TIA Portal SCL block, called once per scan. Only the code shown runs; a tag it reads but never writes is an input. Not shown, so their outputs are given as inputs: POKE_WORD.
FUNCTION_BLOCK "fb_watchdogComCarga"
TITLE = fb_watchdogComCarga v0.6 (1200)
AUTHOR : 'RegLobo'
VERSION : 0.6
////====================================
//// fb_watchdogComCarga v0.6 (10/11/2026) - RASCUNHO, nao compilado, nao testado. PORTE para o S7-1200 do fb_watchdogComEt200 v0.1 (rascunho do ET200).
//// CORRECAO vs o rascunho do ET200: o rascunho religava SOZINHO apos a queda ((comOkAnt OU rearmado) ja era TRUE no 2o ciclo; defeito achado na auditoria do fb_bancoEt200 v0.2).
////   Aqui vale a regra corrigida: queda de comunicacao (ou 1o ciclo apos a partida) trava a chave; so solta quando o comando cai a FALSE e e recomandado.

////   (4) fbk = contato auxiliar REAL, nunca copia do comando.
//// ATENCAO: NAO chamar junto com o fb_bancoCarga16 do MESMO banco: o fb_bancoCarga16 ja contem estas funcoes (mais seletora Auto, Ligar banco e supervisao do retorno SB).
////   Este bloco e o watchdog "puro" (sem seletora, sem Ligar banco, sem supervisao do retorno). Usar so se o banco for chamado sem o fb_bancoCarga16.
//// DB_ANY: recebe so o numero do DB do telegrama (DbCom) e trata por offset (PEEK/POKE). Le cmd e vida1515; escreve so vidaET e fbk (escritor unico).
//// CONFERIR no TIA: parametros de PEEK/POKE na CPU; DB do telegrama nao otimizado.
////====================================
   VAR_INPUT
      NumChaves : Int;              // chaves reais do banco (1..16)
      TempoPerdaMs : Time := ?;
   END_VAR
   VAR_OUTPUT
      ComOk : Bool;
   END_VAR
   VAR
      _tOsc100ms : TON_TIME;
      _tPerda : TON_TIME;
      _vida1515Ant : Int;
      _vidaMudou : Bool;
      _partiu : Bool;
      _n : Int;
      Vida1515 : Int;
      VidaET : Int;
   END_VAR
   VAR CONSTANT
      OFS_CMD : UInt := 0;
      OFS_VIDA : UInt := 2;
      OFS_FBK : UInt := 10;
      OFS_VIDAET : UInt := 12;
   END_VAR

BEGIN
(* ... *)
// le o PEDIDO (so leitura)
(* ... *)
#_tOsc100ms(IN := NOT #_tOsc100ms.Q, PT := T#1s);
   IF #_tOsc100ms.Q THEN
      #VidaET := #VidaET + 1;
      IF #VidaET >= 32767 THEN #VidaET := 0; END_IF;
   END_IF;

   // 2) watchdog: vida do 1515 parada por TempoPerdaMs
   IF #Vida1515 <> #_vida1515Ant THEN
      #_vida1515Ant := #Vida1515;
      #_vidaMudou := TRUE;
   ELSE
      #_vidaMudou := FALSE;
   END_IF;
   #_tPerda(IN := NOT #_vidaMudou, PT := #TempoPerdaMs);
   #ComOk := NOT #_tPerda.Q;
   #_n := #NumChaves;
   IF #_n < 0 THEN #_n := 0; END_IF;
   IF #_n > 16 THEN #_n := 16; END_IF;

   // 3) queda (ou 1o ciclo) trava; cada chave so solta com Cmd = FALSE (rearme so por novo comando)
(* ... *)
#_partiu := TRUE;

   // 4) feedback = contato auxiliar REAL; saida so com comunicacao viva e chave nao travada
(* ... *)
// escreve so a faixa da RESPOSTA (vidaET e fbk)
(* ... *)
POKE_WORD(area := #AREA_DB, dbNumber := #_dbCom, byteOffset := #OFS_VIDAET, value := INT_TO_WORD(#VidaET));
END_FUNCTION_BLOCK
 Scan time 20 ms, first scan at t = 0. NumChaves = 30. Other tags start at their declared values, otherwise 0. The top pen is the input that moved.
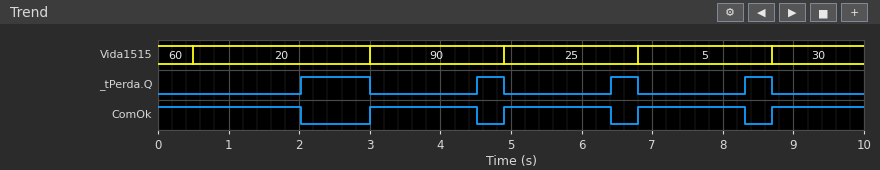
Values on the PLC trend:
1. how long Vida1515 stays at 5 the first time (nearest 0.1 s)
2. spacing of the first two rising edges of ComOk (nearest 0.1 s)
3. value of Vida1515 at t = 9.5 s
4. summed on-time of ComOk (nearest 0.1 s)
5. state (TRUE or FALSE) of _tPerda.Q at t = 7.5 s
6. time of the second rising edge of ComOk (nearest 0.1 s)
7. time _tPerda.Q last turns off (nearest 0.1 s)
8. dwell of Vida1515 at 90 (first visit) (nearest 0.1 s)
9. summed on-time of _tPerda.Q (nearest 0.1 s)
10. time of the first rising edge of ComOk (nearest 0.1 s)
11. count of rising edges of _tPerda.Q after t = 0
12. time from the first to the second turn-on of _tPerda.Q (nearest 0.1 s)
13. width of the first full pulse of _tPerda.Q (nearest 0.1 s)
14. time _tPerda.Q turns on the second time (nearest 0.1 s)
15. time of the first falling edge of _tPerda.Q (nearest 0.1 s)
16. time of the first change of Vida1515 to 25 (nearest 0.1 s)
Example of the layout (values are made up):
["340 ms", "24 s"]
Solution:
["1.9 s", "1.9 s", "30", "7.9 s", "FALSE", "4.9 s", "8.7 s", "1.9 s", "2.1 s", "3.0 s", "4", "2.5 s", "1.0 s", "4.5 s", "3.0 s", "4.9 s"]
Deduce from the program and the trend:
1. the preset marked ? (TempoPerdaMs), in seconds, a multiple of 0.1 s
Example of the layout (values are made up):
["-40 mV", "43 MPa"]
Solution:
["1.5 s"]
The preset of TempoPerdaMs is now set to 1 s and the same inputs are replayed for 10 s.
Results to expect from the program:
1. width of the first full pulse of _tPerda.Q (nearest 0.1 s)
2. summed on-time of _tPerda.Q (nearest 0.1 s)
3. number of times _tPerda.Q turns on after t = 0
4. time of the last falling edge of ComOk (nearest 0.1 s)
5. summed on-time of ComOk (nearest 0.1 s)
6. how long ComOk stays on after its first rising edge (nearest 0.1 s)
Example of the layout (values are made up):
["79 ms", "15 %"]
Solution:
["1.5 s", "4.4 s", "5", "9.7 s", "5.6 s", "1.0 s"]
